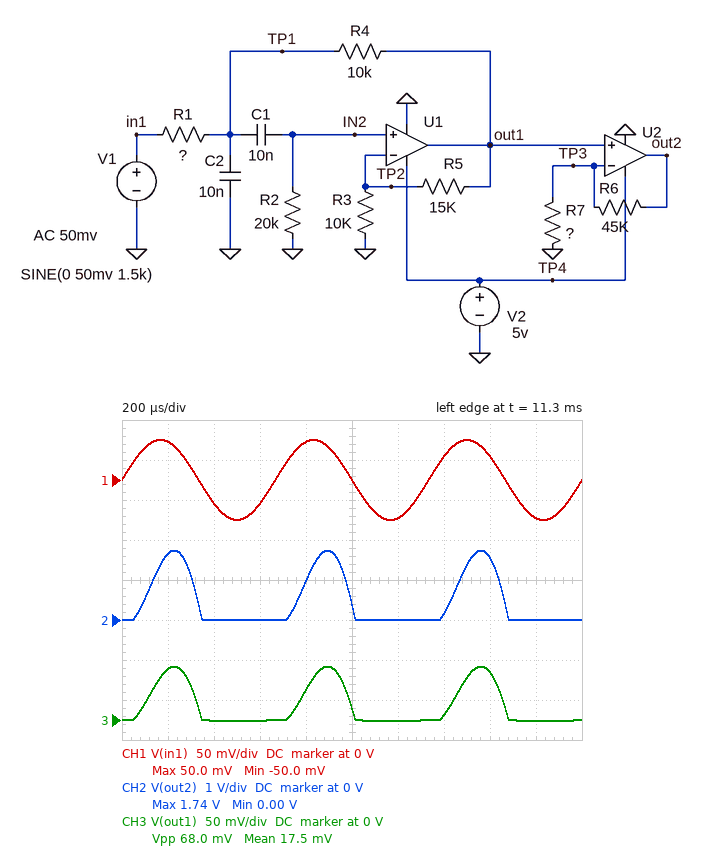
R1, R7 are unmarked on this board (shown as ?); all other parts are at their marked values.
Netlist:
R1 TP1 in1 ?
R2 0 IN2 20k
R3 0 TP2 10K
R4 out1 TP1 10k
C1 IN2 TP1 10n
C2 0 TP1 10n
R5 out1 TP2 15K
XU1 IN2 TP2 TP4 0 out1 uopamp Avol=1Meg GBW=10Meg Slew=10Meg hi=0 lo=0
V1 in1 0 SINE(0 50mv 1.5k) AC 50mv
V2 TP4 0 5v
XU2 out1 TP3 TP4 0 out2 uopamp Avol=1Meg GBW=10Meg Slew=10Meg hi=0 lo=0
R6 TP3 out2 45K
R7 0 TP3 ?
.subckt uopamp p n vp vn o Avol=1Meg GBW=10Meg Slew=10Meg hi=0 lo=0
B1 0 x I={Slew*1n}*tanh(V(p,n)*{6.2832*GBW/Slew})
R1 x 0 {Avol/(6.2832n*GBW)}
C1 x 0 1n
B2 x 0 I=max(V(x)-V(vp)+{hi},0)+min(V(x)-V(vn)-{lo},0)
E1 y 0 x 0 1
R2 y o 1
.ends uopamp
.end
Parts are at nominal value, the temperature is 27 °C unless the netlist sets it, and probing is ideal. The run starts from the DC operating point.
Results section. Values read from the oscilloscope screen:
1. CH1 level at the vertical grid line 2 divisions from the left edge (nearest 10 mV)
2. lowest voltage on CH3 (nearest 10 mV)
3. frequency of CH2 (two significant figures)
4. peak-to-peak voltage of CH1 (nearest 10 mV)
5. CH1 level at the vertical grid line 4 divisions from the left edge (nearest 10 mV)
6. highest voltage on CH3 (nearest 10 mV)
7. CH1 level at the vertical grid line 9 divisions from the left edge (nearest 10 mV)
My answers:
-30 mV
0 V
1.5 kHz
100 mV
50 mV
70 mV
-50 mV
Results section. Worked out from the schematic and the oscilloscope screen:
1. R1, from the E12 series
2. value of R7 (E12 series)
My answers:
18 kΩ
1.8 kΩ
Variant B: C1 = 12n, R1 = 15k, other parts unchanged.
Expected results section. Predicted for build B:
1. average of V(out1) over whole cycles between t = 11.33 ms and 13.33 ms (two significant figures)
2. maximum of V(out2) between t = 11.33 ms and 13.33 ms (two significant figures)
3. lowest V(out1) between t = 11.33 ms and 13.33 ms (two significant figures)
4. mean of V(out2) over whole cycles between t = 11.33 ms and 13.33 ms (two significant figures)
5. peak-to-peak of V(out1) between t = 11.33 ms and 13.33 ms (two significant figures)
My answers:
20 mV
2.0 V
-1.4 mV
540 mV
78 mV
